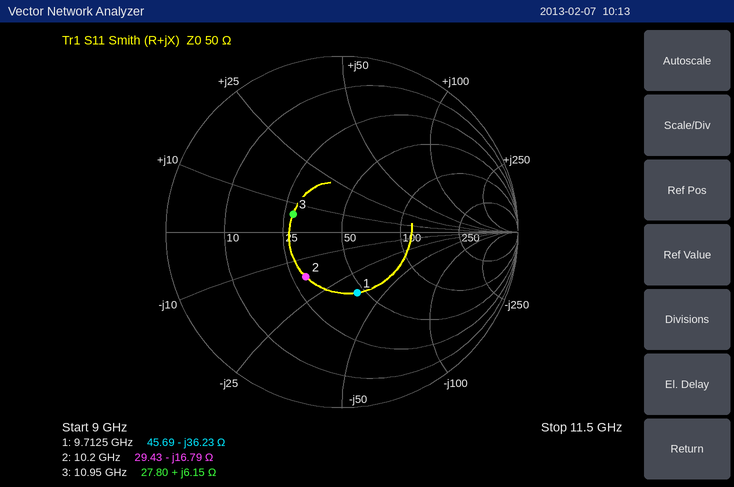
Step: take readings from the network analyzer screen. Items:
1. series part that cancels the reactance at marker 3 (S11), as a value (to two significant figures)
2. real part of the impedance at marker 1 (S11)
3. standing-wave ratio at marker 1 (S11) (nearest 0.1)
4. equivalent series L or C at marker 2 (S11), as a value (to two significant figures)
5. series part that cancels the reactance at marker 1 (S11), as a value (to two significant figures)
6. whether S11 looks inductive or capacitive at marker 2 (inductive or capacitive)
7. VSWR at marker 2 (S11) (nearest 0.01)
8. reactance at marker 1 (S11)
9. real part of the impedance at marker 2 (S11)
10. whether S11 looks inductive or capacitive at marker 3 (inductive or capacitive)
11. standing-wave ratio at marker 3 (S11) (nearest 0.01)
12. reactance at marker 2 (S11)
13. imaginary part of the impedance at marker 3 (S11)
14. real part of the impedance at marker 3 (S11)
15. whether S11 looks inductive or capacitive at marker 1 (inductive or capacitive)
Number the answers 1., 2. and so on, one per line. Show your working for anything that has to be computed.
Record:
1. C = 1/(2π × 10.95 GHz × 6.15 Ω) ≈ 2.4 pF
2. 45.69 Ω
3. 2.1
4. C = 1/(2π × 10.2 GHz × 16.79 Ω) ≈ 929 fF, so 930 fF to two significant figures
5. L = 36.23 Ω/(2π × 9.7125 GHz) ≈ 594 pH, so 590 pH to two significant figures
6. capacitive
7. 1.97
8. -36.23 Ω
9. 29.43 Ω
10. inductive
11. 1.84
12. -16.79 Ω
13. +6.15 Ω
14. 27.80 Ω
15. capacitive
